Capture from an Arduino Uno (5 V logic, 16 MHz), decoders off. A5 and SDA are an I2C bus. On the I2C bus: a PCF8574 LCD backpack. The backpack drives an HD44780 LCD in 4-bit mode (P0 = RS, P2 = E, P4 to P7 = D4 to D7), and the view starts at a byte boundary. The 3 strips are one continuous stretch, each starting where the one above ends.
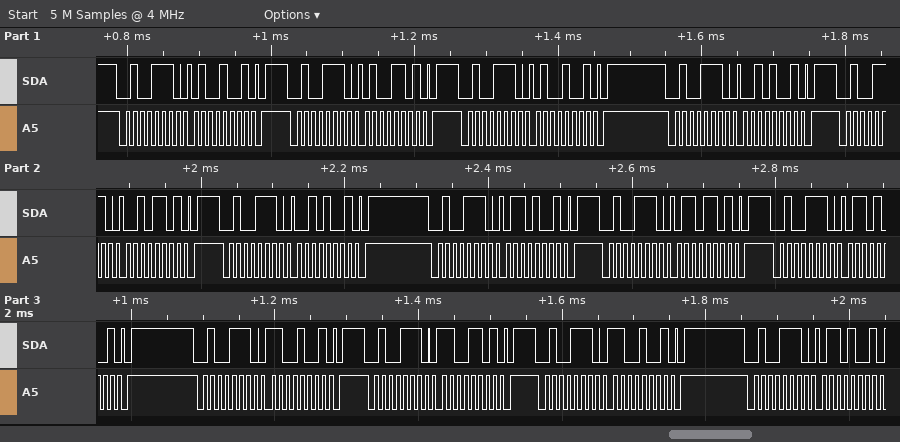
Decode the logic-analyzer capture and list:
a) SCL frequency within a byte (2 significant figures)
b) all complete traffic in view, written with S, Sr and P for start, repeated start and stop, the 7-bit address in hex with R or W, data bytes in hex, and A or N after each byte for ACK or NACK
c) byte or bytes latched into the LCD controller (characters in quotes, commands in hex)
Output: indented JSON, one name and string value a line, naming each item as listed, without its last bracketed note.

{
  "SCL frequency within a byte": "100 kHz",
  "all complete traffic in view, written with S, Sr and P for start, repeated start and stop, the 7-bit address in hex with R or W, data bytes in hex, and A or N after each byte for ACK or NACK": "S 27W A 49 A P S 27W A 4D A P S 27W A 49 A P S 27W A 29 A P S 27W A 2D A P S 27W A 29 A P S 27W A 69 A P S 27W A 6D A P S 27W A 69 A P S 27W A C9 A P S 27W A CD A P S 27W A C9 A P S 27W A 69 A",
  "byte or bytes latched into the LCD controller": "'B' 'l'"
}
